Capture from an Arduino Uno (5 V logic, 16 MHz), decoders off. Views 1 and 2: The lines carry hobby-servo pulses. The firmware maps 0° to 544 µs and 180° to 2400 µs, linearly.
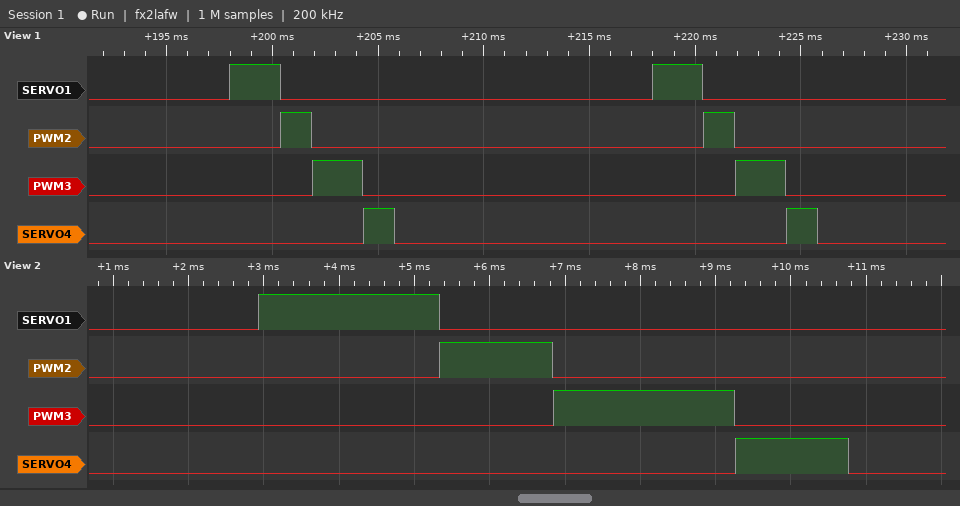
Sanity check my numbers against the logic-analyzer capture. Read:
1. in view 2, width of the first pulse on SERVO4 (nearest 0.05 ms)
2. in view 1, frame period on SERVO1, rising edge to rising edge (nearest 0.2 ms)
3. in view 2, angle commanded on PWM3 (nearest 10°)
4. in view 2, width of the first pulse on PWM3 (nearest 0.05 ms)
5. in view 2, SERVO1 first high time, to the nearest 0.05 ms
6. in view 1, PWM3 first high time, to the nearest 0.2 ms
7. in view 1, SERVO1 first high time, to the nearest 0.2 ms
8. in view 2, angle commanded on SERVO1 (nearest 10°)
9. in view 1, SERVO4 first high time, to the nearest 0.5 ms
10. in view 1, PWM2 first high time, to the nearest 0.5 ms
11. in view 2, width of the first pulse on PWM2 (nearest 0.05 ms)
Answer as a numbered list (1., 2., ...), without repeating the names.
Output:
1. 1.50 ms
2. 20.0 ms
3. 180°
4. 2.40 ms
5. 2.40 ms
6. 2.4 ms
7. 2.4 ms
8. 180°
9. 1.5 ms
10. 1.5 ms
11. 1.50 ms
